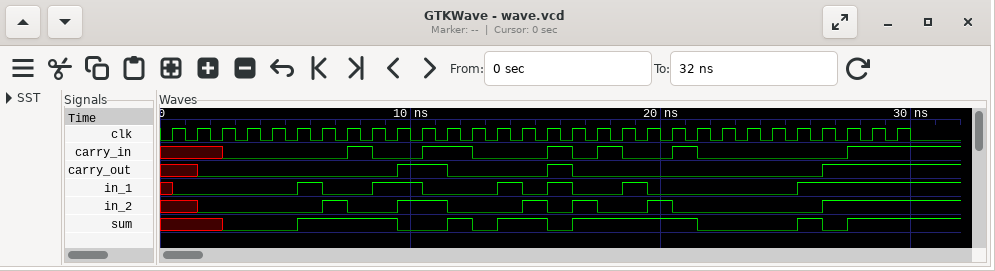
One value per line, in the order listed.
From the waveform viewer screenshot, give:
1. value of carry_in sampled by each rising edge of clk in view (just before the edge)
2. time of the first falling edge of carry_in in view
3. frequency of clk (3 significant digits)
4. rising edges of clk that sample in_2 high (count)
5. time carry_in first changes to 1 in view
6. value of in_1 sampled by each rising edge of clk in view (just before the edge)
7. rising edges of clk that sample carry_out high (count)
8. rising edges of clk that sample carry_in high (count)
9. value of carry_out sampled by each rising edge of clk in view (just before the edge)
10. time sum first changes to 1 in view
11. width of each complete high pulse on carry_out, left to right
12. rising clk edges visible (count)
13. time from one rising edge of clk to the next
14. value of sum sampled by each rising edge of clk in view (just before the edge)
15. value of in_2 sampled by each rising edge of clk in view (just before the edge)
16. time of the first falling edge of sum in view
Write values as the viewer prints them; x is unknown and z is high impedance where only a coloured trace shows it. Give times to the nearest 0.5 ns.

x x x 0 0 0 0 0 1 0 0 1 1 0 0 0 1 0 1 0 0 1 0 0 0 0 0 0 1 1
8.5 ns
1.00 GHz
9
7.5 ns
x 0 0 0 0 0 1 0 0 1 1 0 0 0 1 0 1 0 0 1 0 0 0 0 0 0 1 1 1 1
6
8
x x 0 0 0 0 0 0 0 0 1 1 0 0 0 0 1 0 0 0 0 0 0 0 0 0 0 1 1 1
5.5 ns
2 ns, 1 ns
30
1 ns
x x x 0 0 0 1 1 1 1 0 0 1 0 1 1 0 1 1 1 1 1 0 0 0 0 1 0 1 1
x x 0 0 0 0 0 1 0 0 1 1 0 0 0 1 0 1 0 0 1 0 0 0 0 0 0 1 1 1
9.5 ns
